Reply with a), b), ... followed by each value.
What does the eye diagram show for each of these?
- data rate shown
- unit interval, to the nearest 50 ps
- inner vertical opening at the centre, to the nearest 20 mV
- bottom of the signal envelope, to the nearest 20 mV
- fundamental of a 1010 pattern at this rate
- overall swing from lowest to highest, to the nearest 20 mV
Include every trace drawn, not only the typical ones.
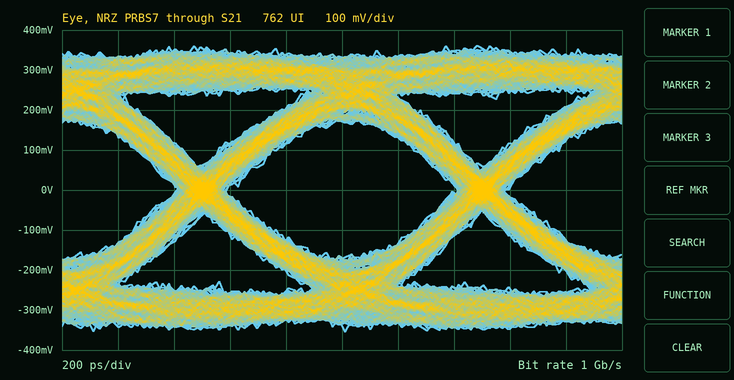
a) 1 Gb/s
b) 1.00 ns
c) 340 mV
d) -360 mV
e) 500 MHz
f) 720 mV
